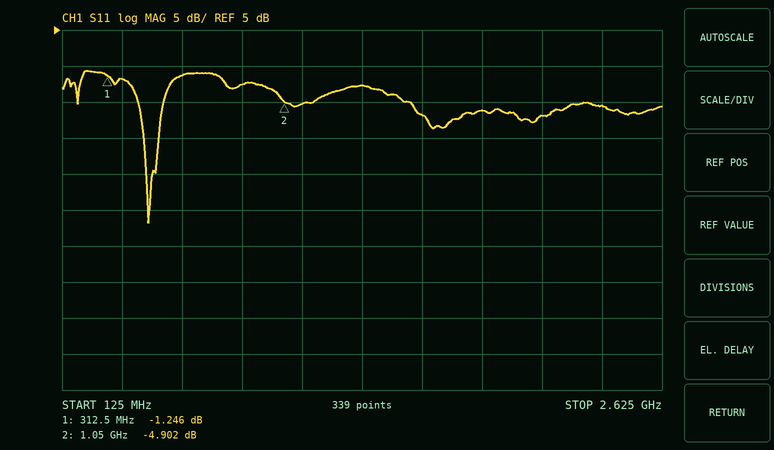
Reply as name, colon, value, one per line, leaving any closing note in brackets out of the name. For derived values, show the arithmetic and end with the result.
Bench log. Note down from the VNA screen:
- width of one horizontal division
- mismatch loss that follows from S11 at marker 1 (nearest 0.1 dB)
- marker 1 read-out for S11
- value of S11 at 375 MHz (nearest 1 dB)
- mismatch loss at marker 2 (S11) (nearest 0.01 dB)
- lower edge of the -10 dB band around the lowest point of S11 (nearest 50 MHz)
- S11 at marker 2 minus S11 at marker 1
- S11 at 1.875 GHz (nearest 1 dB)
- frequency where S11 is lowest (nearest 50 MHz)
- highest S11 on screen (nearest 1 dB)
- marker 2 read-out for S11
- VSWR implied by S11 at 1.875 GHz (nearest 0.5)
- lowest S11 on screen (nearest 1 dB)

width of one horizontal division: 250 MHz
mismatch loss that follows from S11 at marker 1: −10 log10(1 − 10^(-1.246/10)) ≈ 6.0 dB
marker 1 read-out for S11: -1.246 dB
value of S11 at 375 MHz: -2 dB
mismatch loss at marker 2 (S11): −10 log10(1 − 10^(-4.902/10)) ≈ 1.70 dB
lower edge of the -10 dB band around the lowest point of S11: 450 MHz
S11 at marker 2 minus S11 at marker 1: -4.902 − (-1.246) = -3.656 dB
S11 at 1.875 GHz: -6 dB
frequency where S11 is lowest: 500 MHz
highest S11 on screen: -1 dB
marker 2 read-out for S11: -4.902 dB
VSWR implied by S11 at 1.875 GHz: |Γ| = 10^(-6/20) = 0.5012; VSWR = (1 + 0.5012)/(1 − 0.5012) ≈ 3.0
lowest S11 on screen: -22 dB
